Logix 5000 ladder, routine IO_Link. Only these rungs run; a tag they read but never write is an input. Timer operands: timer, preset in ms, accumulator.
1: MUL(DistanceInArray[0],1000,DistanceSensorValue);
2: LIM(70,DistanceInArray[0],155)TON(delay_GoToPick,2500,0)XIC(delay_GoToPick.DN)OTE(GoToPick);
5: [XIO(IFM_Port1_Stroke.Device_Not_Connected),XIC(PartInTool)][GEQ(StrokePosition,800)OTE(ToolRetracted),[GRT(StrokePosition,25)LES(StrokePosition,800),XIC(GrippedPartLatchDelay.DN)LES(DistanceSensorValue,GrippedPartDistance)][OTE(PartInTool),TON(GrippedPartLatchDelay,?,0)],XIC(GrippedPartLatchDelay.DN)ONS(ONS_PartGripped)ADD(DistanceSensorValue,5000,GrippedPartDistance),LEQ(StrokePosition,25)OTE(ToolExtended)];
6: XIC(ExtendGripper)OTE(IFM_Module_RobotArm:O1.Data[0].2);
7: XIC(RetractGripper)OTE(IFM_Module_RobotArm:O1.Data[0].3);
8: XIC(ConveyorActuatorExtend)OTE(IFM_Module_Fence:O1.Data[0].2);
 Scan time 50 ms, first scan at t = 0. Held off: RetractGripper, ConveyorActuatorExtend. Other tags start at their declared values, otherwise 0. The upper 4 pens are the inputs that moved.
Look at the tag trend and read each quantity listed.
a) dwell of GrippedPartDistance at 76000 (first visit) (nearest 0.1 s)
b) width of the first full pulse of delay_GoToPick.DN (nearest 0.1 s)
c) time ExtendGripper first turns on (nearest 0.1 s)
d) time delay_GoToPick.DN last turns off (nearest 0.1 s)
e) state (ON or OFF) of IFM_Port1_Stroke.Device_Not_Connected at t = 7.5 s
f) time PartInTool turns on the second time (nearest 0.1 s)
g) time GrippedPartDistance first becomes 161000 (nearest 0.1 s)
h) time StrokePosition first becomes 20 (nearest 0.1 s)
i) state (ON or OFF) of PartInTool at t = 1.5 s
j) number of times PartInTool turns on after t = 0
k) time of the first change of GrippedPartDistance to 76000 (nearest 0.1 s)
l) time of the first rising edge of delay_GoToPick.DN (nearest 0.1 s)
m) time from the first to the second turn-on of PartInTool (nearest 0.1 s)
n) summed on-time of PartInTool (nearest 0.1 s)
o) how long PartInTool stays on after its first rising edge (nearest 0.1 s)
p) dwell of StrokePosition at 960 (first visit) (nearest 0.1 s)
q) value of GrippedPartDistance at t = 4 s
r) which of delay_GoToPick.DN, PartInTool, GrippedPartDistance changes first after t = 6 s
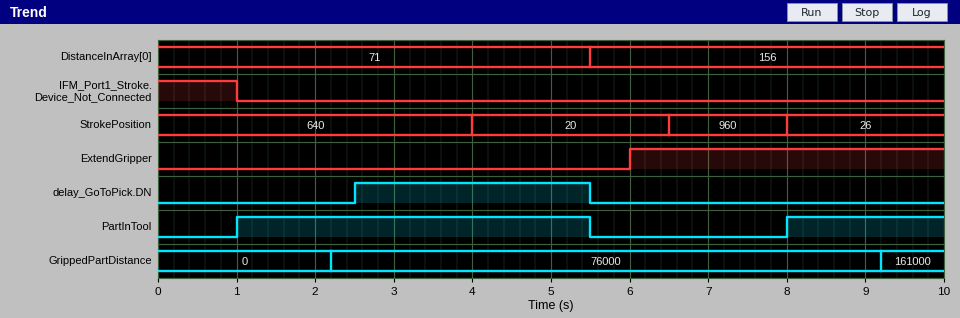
7.0 s
3.0 s
6.0 s
5.5 s
OFF
8.0 s
9.2 s
4.0 s
ON
2
2.2 s
2.5 s
7.0 s
6.5 s
4.5 s
1.5 s
76000
PartInTool
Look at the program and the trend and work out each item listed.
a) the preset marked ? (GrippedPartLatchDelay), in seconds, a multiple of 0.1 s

1.2 s
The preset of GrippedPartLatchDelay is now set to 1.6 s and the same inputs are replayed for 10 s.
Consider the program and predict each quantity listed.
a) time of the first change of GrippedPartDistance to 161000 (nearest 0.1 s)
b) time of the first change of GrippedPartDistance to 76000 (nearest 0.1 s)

9.6 s
2.6 s
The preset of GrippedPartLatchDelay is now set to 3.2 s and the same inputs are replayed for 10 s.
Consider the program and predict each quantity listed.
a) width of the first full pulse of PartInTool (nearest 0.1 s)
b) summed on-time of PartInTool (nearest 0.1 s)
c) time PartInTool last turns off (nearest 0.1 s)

3.0 s
5.0 s
4.0 s
